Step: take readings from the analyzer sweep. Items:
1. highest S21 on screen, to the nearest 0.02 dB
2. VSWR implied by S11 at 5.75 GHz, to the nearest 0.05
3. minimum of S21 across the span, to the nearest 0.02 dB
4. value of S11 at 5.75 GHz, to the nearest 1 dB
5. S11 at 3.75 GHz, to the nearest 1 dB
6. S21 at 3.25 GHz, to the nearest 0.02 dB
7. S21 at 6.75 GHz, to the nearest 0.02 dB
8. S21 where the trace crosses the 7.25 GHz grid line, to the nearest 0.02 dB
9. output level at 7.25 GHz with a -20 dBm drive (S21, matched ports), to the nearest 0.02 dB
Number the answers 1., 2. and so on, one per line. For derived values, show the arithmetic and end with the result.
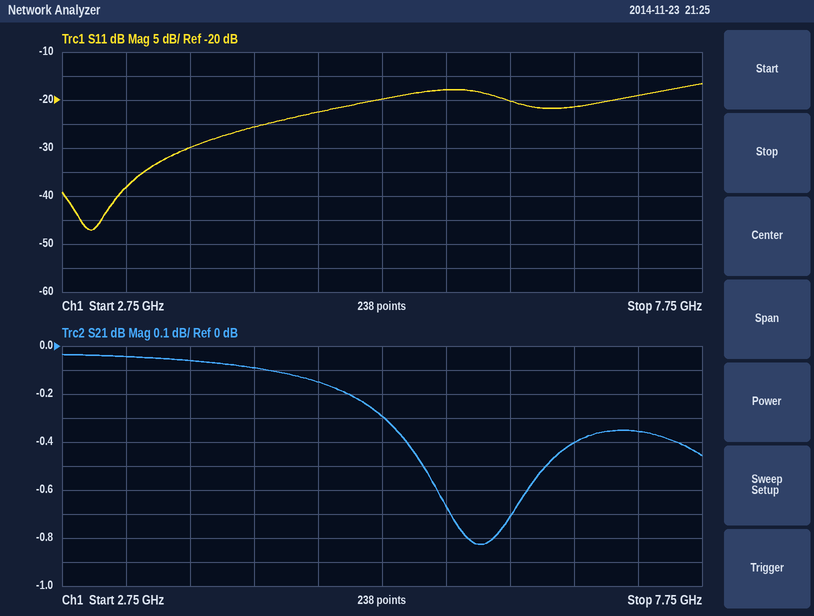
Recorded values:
1. -0.04 dB
2. |Γ| = 10^(-18/20) = 0.1259; VSWR = (1 + 0.1259)/(1 − 0.1259) ≈ 1.29, so 1.30 to the nearest 0.05
3. -0.82 dB
4. -18 dB
5. -30 dB
6. -0.04 dB
7. -0.40 dB
8. -0.36 dB
9. -20 dBm + (-0.36 dB) = -20.36 dBm
